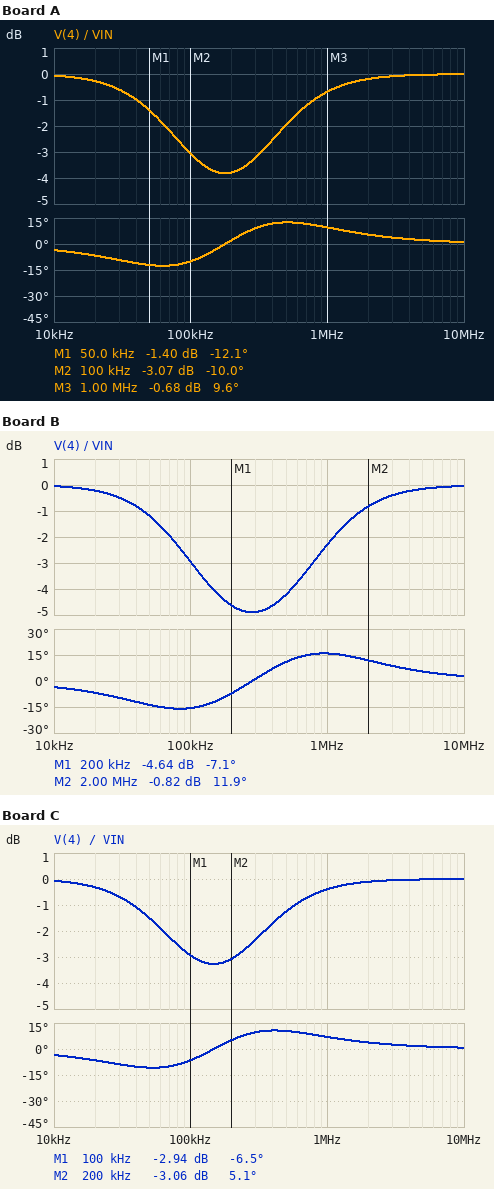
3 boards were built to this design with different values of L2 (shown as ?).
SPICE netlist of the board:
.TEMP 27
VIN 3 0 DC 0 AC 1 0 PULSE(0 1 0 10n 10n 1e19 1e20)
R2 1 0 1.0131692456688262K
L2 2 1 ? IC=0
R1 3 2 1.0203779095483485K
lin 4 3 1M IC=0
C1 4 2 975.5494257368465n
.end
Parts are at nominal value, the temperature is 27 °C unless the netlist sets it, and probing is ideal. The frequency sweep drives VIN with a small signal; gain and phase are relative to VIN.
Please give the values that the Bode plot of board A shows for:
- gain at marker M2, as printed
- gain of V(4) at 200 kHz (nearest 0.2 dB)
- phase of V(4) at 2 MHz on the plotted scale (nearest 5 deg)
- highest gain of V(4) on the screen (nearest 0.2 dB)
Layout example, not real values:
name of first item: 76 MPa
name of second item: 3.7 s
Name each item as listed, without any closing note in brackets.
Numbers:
gain at marker M2, as printed: -3.07 dB
gain of V(4) at 200 kHz: -3.8 dB
phase of V(4) at 2 MHz on the plotted scale: 5 deg
highest gain of V(4) on the screen: 0 dB
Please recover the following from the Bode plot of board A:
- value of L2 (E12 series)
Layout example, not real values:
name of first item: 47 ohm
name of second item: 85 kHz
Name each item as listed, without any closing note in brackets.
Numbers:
value of L2: 820 µH
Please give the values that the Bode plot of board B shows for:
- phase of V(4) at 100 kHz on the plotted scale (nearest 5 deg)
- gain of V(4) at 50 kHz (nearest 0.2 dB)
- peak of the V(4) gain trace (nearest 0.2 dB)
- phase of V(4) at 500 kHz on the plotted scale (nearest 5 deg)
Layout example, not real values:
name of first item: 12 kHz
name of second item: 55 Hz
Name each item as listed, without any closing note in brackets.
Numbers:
phase of V(4) at 100 kHz on the plotted scale: -15 deg
gain of V(4) at 50 kHz: -1.2 dB
peak of the V(4) gain trace: 0 dB
phase of V(4) at 500 kHz on the plotted scale: 10 deg
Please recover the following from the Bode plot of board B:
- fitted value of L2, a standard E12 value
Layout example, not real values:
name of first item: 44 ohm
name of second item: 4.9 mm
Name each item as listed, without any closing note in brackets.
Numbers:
fitted value of L2, a standard E12 value: 330 µH
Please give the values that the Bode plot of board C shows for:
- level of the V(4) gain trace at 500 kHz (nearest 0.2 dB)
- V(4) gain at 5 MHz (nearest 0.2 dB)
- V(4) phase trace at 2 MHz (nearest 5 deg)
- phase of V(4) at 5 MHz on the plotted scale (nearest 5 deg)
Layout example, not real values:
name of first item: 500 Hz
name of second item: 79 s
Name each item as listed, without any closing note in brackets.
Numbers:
level of the V(4) gain trace at 500 kHz: -1.2 dB
V(4) gain at 5 MHz: 0 dB
V(4) phase trace at 2 MHz: 5 deg
phase of V(4) at 5 MHz on the plotted scale: 0 deg
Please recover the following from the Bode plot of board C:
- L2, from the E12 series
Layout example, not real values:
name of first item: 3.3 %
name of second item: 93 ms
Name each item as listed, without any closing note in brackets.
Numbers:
L2, from the E12 series: 1.2 mH
